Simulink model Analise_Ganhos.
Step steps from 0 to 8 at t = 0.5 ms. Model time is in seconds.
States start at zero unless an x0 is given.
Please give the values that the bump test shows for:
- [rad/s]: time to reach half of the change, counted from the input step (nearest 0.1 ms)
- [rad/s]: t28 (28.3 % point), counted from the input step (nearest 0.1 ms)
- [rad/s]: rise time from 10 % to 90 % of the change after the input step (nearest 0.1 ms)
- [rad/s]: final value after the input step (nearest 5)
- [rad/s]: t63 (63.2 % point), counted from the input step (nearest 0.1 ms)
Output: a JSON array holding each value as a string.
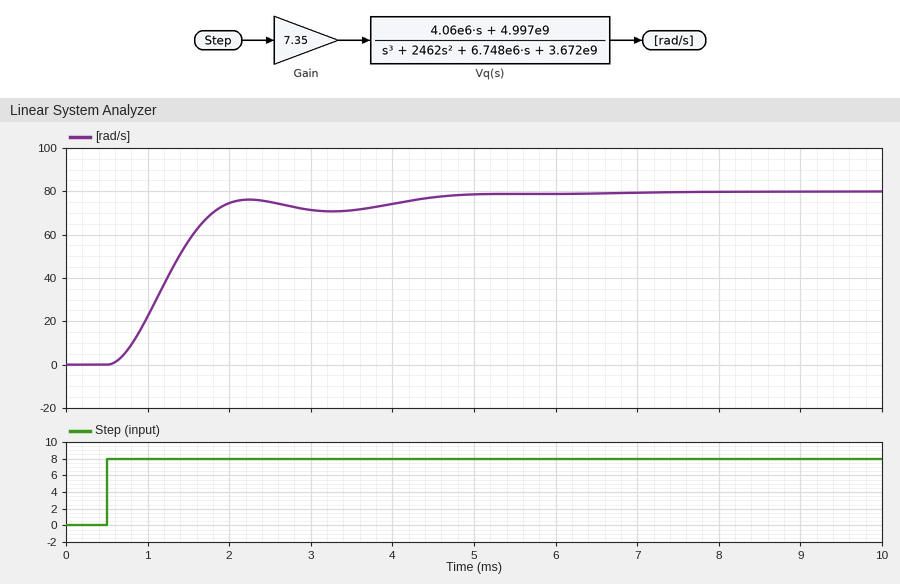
["0.7 ms", "0.5 ms", "1.1 ms", "80", "0.9 ms"]
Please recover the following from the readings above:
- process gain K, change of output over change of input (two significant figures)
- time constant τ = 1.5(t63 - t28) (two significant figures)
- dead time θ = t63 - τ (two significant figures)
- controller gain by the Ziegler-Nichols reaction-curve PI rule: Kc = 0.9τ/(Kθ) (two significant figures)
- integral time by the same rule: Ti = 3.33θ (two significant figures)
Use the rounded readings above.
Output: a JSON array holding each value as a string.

["10", "0.60 ms", "0.30 ms", "0.18", "1.00 ms"]
